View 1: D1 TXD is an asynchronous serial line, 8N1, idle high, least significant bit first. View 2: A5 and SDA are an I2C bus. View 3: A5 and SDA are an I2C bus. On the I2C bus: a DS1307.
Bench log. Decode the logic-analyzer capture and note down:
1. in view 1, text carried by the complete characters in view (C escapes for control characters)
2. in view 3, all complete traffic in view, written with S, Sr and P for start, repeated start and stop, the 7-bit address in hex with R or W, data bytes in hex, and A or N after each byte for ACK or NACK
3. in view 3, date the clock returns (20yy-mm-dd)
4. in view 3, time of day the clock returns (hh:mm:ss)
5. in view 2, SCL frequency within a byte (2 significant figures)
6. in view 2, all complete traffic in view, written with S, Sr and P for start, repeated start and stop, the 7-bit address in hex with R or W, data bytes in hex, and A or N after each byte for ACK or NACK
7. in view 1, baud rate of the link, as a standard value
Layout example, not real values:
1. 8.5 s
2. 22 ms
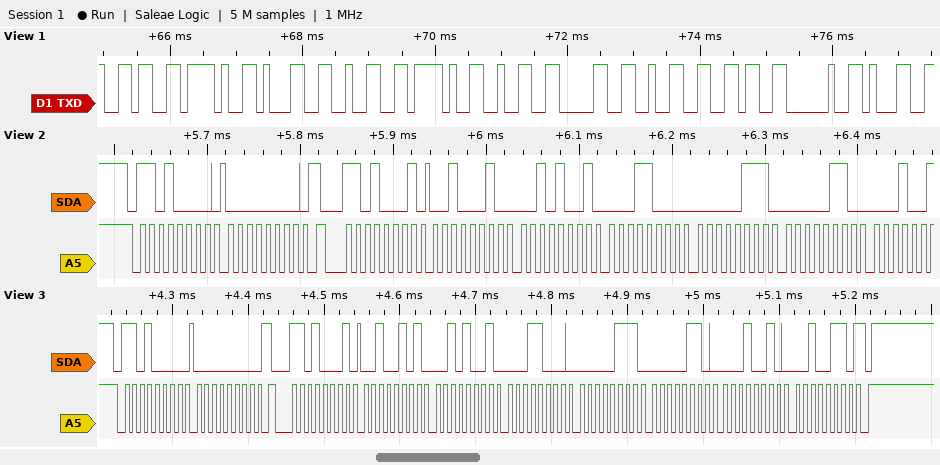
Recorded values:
1. "6/12/2026 1"
2. S 68W A 00 A Sr 68R A 25 A 29 A 18 A 07 A 06 A 12 A 26 N P
3. 2026-12-06
4. 18:29:25
5. 100 kHz
6. S 68W A 00 A Sr 68R A 22 A 29 A 18 A 07 A 06 A
7. 9600 baud
